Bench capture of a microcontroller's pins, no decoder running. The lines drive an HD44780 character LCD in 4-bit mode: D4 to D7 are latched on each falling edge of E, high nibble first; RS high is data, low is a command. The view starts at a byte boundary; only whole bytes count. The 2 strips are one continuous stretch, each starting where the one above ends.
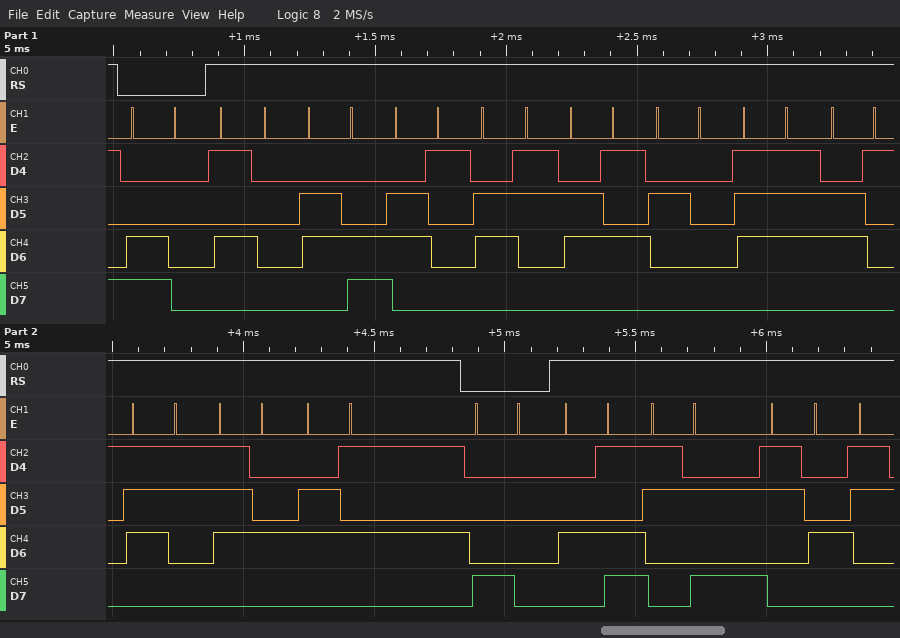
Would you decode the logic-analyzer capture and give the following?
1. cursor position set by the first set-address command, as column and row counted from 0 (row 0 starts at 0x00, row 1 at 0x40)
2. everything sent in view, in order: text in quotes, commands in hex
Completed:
column 0, row 1
0xC0 "Place waste" 0x80 "M:4"
